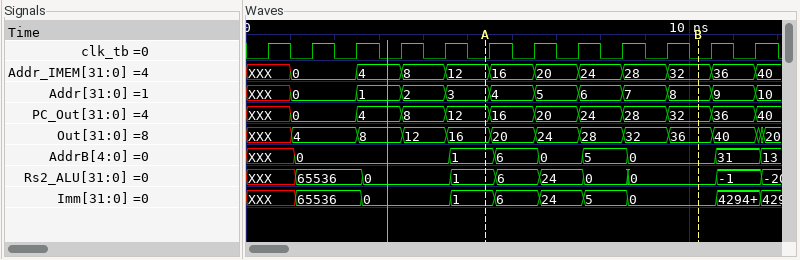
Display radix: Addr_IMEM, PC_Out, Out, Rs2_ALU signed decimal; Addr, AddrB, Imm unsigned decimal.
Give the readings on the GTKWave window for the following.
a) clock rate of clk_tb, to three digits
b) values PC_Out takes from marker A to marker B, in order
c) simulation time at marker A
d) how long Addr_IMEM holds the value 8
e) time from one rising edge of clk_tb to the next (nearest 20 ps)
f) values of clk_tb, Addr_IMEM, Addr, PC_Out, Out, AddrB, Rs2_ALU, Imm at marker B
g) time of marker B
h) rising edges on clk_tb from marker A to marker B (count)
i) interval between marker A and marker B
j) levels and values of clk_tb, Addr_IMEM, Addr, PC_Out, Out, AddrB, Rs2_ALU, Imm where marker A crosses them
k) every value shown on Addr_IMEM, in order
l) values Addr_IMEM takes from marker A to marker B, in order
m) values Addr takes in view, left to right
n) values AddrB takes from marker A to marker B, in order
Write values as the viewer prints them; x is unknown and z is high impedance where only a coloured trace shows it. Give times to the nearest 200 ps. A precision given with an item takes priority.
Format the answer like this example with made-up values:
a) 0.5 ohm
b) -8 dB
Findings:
a) 1.00 GHz
b) 12, 16, 20, 24, 28, 32
c) 5400 ps
d) 1000 ps
e) 1000 ps
f) clk_tb=0, Addr_IMEM=32, Addr=8, PC_Out=32, Out=36, AddrB=0, Rs2_ALU=0, Imm=0
g) 10200 ps
h) 5
i) 4800 ps
j) clk_tb=0, Addr_IMEM=12, Addr=3, PC_Out=12, Out=16, AddrB=1, Rs2_ALU=1, Imm=1
k) XXX, 0, 4, 8, 12, 16, 20, 24, 28, 32, 36, 40
l) 12, 16, 20, 24, 28, 32
m) XXX, 0, 1, 2, 3, 4, 5, 6, 7, 8, 9, 10
n) 1, 6, 0, 5, 0
